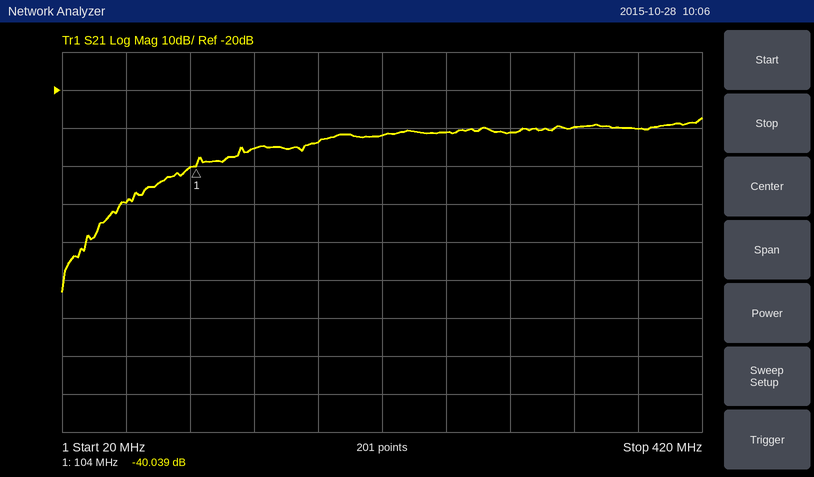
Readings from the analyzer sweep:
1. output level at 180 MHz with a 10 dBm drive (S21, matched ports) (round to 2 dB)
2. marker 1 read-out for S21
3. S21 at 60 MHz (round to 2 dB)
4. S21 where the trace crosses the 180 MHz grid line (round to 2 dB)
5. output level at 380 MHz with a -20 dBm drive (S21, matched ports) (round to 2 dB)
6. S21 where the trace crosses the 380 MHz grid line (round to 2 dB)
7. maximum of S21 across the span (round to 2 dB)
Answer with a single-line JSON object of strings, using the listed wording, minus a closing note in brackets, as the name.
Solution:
{"output level at 180 MHz with a 10 dBm drive (S21, matched ports)": "-24 dBm", "marker 1 read-out for S21": "-40.039 dB", "S21 at 60 MHz": "-50 dB", "S21 where the trace crosses the 180 MHz grid line": "-34 dB", "output level at 380 MHz with a -20 dBm drive (S21, matched ports)": "-50 dBm", "S21 where the trace crosses the 380 MHz grid line": "-30 dB", "maximum of S21 across the span": "-28 dB"}
